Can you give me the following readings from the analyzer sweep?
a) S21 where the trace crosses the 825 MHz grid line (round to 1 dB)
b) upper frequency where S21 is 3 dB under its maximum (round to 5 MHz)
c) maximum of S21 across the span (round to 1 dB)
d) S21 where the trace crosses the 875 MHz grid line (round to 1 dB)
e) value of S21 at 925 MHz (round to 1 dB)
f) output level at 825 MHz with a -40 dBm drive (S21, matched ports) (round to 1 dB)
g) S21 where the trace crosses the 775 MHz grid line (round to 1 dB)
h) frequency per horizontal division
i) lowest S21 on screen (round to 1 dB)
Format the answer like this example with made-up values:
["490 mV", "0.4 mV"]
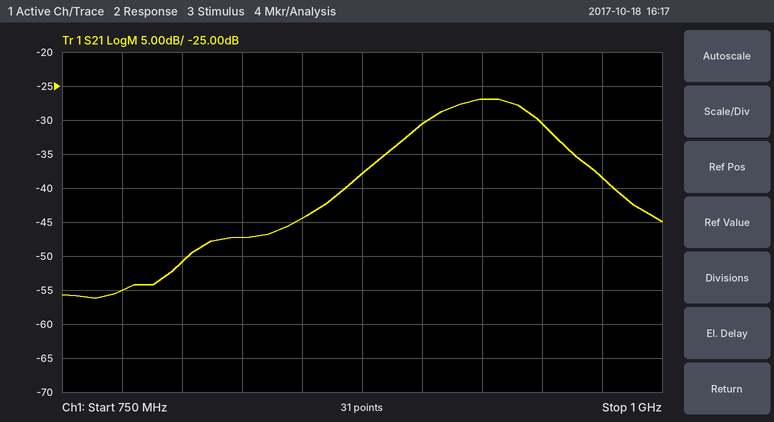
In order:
["-47 dB", "950 MHz", "-27 dB", "-38 dB", "-27 dB", "-87 dBm", "-55 dB", "25 MHz", "-56 dB"]
